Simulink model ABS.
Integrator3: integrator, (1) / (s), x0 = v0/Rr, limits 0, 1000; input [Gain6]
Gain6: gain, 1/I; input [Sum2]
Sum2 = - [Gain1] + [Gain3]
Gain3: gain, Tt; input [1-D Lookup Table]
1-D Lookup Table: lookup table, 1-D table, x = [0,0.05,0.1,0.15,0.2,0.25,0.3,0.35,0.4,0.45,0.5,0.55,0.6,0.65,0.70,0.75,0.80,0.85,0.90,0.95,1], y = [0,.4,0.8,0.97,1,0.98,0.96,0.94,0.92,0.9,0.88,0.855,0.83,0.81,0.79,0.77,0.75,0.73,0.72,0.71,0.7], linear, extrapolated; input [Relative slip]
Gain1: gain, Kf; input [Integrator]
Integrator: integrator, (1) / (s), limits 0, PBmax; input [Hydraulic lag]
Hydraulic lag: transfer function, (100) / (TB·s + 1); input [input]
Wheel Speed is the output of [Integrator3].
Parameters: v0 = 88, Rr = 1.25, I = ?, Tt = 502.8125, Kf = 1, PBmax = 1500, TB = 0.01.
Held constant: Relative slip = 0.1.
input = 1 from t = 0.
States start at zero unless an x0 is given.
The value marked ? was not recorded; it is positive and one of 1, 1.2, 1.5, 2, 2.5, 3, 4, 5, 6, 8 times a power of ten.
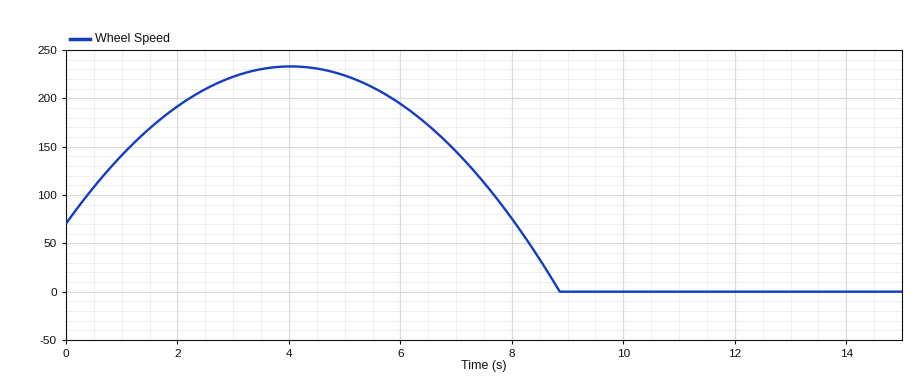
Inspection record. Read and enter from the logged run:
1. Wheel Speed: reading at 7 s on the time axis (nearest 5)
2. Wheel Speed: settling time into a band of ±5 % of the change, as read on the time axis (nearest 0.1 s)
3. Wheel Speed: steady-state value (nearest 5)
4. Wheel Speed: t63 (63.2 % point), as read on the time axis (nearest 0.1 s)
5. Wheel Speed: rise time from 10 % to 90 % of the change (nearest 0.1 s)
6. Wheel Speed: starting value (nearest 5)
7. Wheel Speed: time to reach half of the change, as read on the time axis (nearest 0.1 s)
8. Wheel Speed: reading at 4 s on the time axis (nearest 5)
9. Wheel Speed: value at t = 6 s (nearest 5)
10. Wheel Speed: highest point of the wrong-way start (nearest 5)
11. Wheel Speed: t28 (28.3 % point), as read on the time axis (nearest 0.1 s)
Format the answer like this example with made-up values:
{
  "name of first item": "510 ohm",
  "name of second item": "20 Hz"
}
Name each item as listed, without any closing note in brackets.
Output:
{
  "Wheel Speed: reading at 7 s on the time axis": "145",
  "Wheel Speed: settling time into a band of ±5 % of the change, as read on the time axis": "8.8 s",
  "Wheel Speed: steady-state value": "0",
  "Wheel Speed: t63 (63.2 % point), as read on the time axis": "8.6 s",
  "Wheel Speed: rise time from 10 % to 90 % of the change": "0.6 s",
  "Wheel Speed: starting value": "70",
  "Wheel Speed: time to reach half of the change, as read on the time axis": "8.5 s",
  "Wheel Speed: reading at 4 s on the time axis": "235",
  "Wheel Speed: value at t = 6 s": "195",
  "Wheel Speed: highest point of the wrong-way start": "235",
  "Wheel Speed: t28 (28.3 % point), as read on the time axis": "8.3 s"
}
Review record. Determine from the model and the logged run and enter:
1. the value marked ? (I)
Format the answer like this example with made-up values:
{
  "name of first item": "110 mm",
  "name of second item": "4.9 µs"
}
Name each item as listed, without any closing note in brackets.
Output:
{
  "the value marked ?": "5"
}
